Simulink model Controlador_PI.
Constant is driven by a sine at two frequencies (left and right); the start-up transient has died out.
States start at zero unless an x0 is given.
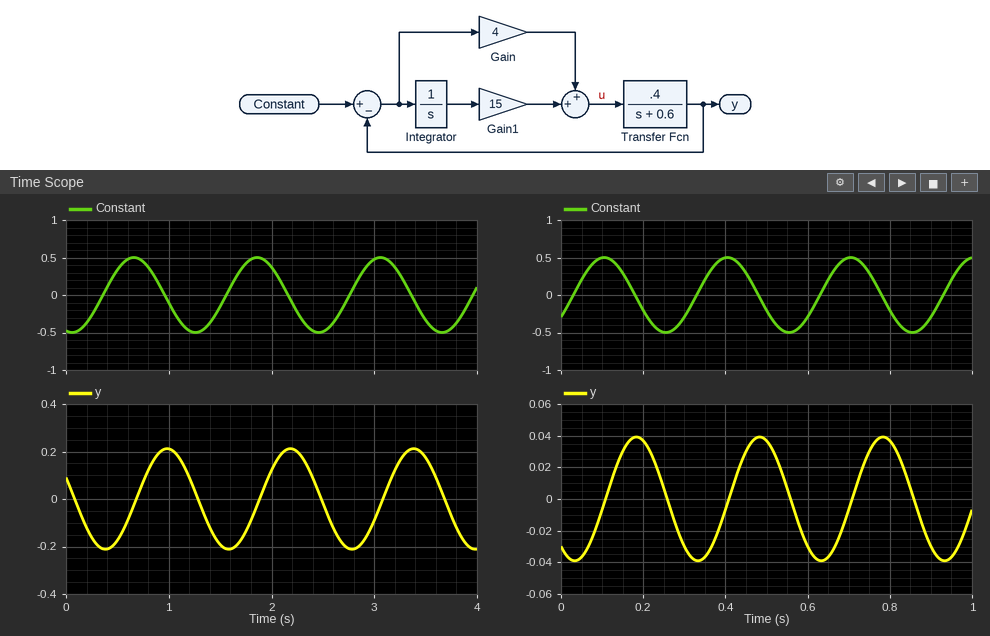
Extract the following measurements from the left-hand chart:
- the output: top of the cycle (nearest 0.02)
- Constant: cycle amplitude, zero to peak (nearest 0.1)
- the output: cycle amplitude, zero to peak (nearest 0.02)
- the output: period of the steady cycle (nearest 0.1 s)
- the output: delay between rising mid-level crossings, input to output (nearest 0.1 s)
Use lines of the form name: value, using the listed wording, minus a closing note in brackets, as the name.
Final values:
the output: top of the cycle: 0.22
Constant: cycle amplitude, zero to peak: 0.5
the output: cycle amplitude, zero to peak: 0.22
the output: period of the steady cycle: 1.2 s
the output: delay between rising mid-level crossings, input to output: 0.3 s
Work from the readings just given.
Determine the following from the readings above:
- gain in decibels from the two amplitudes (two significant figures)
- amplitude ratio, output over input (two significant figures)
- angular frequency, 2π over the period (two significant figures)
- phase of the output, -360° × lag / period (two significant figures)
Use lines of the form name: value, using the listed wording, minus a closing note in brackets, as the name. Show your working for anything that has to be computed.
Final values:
gain in decibels from the two amplitudes: 20 log10(0.22 / 0.5) = -7.1 dB
amplitude ratio, output over input: 0.22 / 0.5 = 0.44
angular frequency, 2π over the period: 2π / 1.2 = 5.2 rad/s
phase of the output, -360° × lag / period: -360 × 0.3 / 1.2 = -90°
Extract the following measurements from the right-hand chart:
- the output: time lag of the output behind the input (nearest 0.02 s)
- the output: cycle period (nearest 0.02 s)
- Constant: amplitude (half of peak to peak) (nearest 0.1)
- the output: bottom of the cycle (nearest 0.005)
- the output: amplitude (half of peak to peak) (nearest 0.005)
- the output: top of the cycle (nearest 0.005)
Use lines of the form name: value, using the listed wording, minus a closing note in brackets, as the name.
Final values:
the output: time lag of the output behind the input: 0.08 s
the output: cycle period: 0.30 s
Constant: amplitude (half of peak to peak): 0.5
the output: bottom of the cycle: -0.040
the output: amplitude (half of peak to peak): 0.040
the output: top of the cycle: 0.040
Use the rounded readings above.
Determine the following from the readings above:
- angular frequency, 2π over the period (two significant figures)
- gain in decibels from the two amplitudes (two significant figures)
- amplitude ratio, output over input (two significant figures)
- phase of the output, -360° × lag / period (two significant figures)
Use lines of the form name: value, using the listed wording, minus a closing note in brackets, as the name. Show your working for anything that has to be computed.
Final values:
angular frequency, 2π over the period: 2π / 0.3 = 21 rad/s
gain in decibels from the two amplitudes: 20 log10(0.04 / 0.5) = -22 dB
amplitude ratio, output over input: 0.04 / 0.5 = 0.080
phase of the output, -360° × lag / period: -360 × 0.08 / 0.3 = -96°
